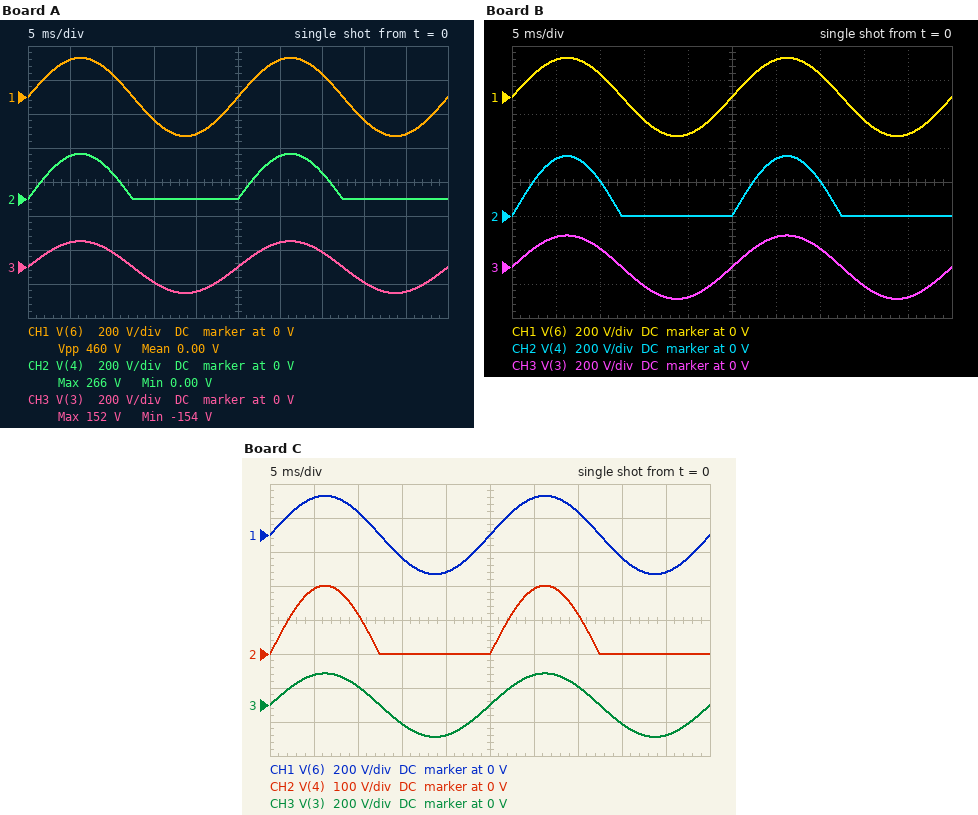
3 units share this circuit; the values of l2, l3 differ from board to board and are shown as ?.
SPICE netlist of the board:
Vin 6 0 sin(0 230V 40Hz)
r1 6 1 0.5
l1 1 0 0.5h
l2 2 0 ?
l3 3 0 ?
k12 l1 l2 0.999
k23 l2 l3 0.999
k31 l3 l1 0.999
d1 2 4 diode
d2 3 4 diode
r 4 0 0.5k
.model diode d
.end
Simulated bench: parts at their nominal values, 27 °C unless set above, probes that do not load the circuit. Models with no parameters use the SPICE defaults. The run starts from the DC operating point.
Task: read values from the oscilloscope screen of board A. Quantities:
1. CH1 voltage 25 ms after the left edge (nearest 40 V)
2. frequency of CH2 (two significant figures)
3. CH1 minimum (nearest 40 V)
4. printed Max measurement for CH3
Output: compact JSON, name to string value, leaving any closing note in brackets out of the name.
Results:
{"CH1 voltage 25 ms after the left edge": "0 V", "frequency of CH2": "40 Hz", "CH1 minimum": "-240 V", "printed Max measurement for CH3": "152 V"}
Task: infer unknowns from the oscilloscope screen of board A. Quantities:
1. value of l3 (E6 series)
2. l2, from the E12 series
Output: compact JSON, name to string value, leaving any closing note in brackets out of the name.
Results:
{"value of l3": "220 mH", "l2, from the E12 series": "680 mH"}
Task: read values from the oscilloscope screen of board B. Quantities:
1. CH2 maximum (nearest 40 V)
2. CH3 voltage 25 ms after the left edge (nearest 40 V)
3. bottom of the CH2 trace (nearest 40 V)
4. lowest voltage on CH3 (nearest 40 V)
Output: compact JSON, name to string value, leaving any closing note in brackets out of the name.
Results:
{"CH2 maximum": "360 V", "CH3 voltage 25 ms after the left edge": "0 V", "bottom of the CH2 trace": "0 V", "lowest voltage on CH3": "-200 V"}
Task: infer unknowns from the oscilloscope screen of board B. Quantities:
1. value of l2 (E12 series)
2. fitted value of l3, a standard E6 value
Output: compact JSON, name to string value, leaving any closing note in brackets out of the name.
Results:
{"value of l2": "1.2 H", "fitted value of l3, a standard E6 value": "330 mH"}
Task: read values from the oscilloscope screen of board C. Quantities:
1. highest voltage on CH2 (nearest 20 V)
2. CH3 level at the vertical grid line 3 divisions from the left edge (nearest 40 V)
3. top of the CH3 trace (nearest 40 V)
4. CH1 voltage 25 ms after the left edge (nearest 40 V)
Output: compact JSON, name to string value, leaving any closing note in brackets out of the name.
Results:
{"highest voltage on CH2": "200 V", "CH3 level at the vertical grid line 3 divisions from the left edge": "-120 V", "top of the CH3 trace": "200 V", "CH1 voltage 25 ms after the left edge": "0 V"}
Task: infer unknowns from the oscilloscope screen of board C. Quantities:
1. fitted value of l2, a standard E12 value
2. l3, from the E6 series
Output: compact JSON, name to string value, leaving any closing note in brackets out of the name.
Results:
{"fitted value of l2, a standard E12 value": "390 mH", "l3, from the E6 series": "330 mH"}
